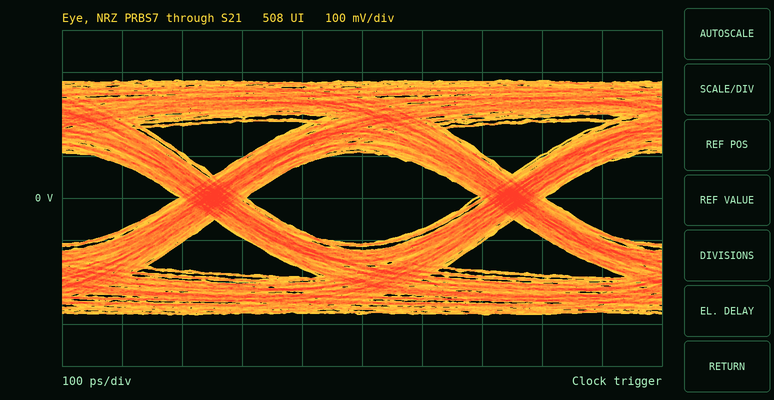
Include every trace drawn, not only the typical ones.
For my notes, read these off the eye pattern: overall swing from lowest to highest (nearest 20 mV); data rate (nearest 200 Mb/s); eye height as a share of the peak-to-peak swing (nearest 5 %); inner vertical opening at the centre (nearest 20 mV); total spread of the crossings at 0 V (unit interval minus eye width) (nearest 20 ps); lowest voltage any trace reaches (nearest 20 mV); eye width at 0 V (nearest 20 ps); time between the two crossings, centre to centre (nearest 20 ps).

560 mV
2.0 Gb/s
40 %
220 mV
120 ps
-280 mV
380 ps
500 ps
